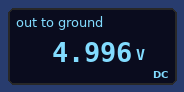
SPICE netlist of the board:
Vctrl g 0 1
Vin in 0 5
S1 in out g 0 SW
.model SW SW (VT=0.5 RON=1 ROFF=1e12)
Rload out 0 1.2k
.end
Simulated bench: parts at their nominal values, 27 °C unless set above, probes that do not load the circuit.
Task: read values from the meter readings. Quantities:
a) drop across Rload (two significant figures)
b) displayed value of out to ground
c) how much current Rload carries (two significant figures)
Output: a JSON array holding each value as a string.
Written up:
["5.0 V", "4.996 V", "4.2 mA"]
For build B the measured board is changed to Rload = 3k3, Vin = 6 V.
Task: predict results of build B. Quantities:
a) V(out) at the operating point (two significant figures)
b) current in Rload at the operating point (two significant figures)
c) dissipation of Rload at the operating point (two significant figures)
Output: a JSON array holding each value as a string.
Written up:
["6.0 V", "1.8 mA", "11 mW"]
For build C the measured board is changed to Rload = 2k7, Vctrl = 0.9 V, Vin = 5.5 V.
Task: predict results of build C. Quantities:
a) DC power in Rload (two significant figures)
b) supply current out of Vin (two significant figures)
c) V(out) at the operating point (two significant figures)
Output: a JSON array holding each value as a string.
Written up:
["11 mW", "2.0 mA", "5.5 V"]
